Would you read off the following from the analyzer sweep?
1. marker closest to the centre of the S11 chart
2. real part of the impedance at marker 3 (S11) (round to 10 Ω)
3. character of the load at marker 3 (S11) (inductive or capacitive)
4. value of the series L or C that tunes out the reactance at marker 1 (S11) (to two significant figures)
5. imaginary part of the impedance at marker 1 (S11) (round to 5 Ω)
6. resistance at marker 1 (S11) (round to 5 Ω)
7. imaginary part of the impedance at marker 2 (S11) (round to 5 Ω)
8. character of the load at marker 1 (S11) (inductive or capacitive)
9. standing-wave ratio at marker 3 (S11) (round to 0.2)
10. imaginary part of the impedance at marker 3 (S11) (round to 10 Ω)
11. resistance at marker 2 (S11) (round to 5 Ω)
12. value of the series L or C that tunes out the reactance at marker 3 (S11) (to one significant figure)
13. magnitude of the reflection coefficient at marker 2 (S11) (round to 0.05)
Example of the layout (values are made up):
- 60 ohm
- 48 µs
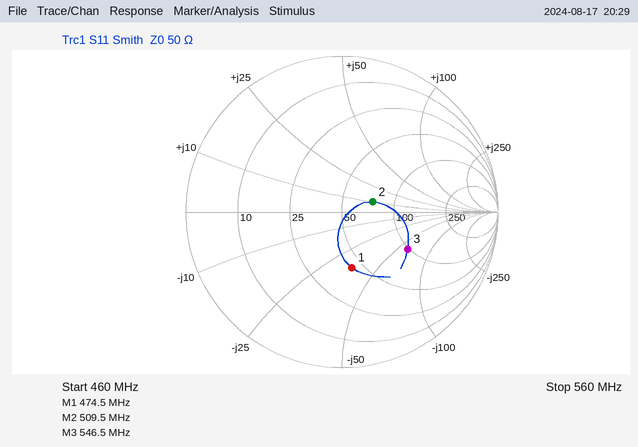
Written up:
- marker 2
- 100 Ω
- capacitive
- 12 nH
- -35 Ω
- 45 Ω
- +10 Ω
- capacitive
- 2.8
- -60 Ω
- 75 Ω
- 20 nH
- 0.20
